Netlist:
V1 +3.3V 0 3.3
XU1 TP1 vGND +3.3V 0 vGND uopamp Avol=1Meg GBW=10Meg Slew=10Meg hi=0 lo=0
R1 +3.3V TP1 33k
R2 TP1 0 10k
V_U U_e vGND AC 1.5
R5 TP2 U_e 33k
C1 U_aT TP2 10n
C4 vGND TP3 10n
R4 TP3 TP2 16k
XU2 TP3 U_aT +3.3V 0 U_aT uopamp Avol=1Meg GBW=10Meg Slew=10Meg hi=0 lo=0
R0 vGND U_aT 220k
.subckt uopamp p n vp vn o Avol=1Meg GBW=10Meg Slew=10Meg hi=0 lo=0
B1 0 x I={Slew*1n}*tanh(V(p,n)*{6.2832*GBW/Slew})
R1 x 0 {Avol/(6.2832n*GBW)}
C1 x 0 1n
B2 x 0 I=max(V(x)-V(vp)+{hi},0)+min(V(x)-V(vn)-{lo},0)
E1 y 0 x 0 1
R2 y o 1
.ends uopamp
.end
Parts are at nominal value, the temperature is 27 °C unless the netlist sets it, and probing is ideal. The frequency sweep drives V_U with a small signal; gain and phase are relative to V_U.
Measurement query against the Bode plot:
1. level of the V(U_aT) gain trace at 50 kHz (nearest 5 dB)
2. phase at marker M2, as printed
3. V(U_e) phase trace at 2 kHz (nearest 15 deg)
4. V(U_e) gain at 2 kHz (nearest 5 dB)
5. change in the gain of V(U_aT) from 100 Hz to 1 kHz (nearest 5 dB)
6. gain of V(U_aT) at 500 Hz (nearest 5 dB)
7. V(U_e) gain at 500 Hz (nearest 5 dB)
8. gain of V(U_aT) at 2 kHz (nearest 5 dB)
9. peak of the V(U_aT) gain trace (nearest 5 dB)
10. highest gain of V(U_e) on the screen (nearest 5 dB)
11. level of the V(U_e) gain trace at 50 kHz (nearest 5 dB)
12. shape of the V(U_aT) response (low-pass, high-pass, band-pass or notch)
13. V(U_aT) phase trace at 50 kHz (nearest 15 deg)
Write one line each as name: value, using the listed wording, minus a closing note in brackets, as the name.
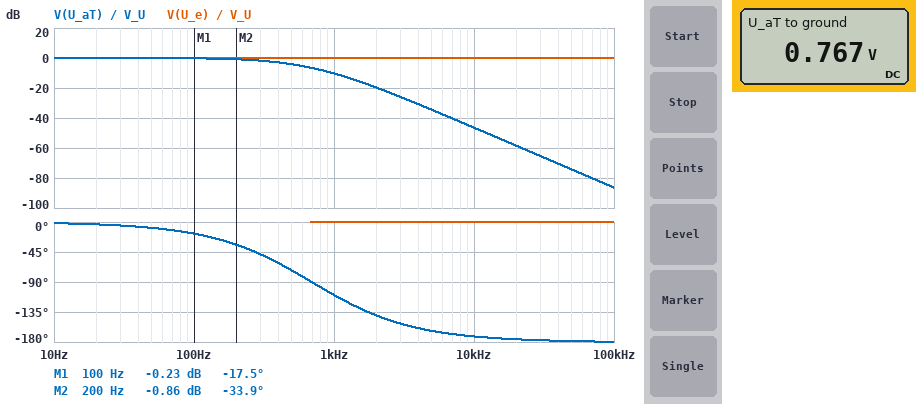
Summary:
level of the V(U_aT) gain trace at 50 kHz: -75 dB
phase at marker M2, as printed: -33.9 deg
V(U_e) phase trace at 2 kHz: 0 deg
V(U_e) gain at 2 kHz: 0 dB
change in the gain of V(U_aT) from 100 Hz to 1 kHz: -10 dB
gain of V(U_aT) at 500 Hz: -5 dB
V(U_e) gain at 500 Hz: 0 dB
gain of V(U_aT) at 2 kHz: -20 dB
peak of the V(U_aT) gain trace: 0 dB
highest gain of V(U_e) on the screen: 0 dB
level of the V(U_e) gain trace at 50 kHz: 0 dB
shape of the V(U_aT) response: low-pass
V(U_aT) phase trace at 50 kHz: -180 deg
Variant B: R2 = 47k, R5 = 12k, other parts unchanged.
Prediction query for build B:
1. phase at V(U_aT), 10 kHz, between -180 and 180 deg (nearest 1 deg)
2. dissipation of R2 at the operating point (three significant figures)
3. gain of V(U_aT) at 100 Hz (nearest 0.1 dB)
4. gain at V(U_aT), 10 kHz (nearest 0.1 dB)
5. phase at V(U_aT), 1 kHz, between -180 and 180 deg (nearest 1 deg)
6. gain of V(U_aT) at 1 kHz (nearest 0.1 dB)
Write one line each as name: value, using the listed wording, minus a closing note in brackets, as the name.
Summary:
phase at V(U_aT), 10 kHz, between -180 and 180 deg: -167 deg
dissipation of R2 at the operating point: 80.0 µW
gain of V(U_aT) at 100 Hz: -0.1 dB
gain at V(U_aT), 10 kHz: -37.7 dB
phase at V(U_aT), 1 kHz, between -180 and 180 deg: -82 deg
gain of V(U_aT) at 1 kHz: -5.0 dB
